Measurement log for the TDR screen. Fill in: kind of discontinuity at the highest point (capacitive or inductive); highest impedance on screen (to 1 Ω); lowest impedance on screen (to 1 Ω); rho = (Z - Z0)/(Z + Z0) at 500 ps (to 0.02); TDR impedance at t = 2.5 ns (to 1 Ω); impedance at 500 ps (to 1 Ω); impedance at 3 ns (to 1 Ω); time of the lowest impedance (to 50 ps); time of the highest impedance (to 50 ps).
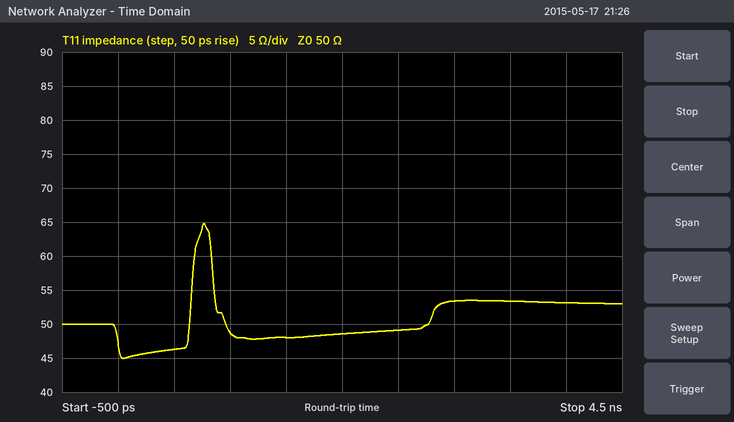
inductive
65 Ω
45 Ω
-0.04
49 Ω
46 Ω
53 Ω
50 ps
750 ps
